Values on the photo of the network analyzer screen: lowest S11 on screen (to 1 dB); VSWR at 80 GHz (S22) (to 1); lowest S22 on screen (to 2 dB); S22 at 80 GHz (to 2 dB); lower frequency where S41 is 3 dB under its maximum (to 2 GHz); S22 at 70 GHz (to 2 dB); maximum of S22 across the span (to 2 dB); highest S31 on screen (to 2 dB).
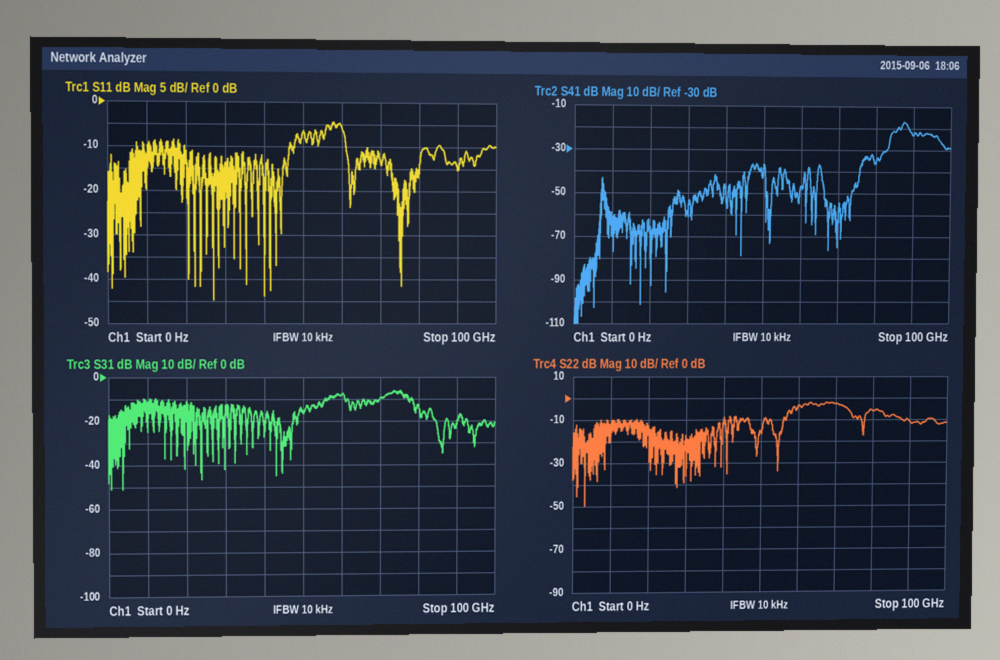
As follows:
-45 dB
3
-50 dB
-6 dB
86 GHz
-2 dB
-2 dB
-6 dB
